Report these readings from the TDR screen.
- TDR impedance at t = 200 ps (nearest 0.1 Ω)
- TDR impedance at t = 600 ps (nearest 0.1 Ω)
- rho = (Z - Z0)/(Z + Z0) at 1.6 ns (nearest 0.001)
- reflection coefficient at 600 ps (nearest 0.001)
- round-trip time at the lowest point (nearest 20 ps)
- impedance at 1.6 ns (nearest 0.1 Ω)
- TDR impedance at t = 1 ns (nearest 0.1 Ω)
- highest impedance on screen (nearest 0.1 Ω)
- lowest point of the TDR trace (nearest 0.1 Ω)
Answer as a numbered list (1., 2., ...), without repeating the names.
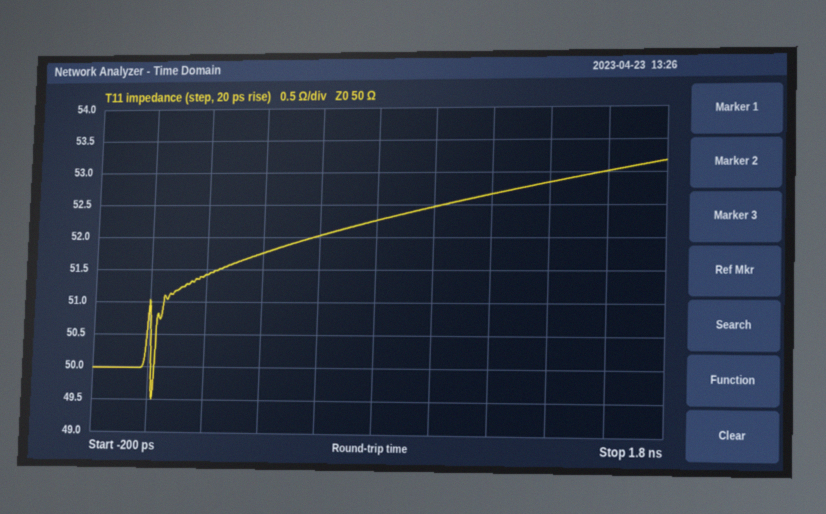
1. 51.4 Ω
2. 52.0 Ω
3. +0.029
4. +0.020
5. 20 ps
6. 53.0 Ω
7. 52.5 Ω
8. 53.2 Ω
9. 49.5 Ω
